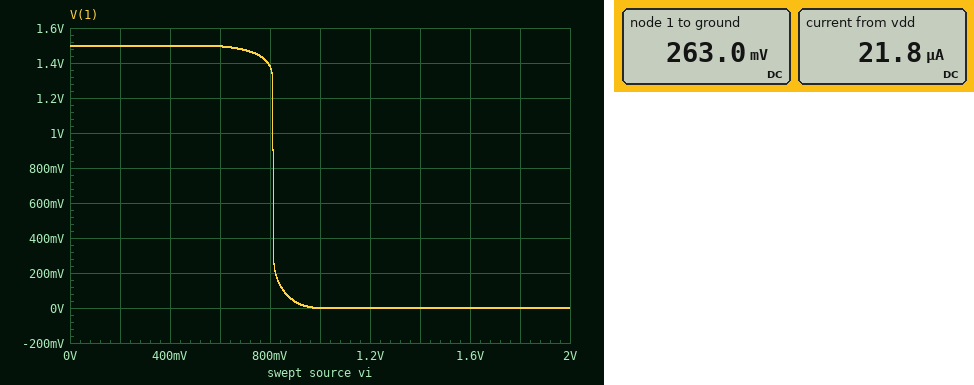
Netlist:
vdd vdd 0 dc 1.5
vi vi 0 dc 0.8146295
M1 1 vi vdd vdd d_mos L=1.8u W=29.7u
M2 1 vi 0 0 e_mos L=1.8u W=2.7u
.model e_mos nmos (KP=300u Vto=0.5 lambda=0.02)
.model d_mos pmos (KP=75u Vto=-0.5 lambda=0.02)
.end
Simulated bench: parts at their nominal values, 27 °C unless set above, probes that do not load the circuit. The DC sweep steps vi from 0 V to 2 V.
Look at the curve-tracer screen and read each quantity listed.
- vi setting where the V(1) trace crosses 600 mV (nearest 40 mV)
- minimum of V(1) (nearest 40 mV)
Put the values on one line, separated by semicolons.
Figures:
800 mV; 0 V
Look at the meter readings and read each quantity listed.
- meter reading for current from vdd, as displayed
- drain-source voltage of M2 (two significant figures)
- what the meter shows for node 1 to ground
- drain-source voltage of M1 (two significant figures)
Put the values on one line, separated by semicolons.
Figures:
21.8 µA; 260 mV; 263.0 mV; -1.2 V
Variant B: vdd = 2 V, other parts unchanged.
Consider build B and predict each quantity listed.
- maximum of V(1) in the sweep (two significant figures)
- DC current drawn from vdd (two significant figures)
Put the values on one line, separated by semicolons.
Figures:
2.0 V; 23 µA
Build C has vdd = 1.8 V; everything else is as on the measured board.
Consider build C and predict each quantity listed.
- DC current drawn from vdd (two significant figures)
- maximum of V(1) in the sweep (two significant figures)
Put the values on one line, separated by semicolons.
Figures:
23 µA; 1.8 V
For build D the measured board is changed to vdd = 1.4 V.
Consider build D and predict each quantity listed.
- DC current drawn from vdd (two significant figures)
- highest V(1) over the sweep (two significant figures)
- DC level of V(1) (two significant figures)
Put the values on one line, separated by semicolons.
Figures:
4.6 µA; 1.4 V; 35 mV
